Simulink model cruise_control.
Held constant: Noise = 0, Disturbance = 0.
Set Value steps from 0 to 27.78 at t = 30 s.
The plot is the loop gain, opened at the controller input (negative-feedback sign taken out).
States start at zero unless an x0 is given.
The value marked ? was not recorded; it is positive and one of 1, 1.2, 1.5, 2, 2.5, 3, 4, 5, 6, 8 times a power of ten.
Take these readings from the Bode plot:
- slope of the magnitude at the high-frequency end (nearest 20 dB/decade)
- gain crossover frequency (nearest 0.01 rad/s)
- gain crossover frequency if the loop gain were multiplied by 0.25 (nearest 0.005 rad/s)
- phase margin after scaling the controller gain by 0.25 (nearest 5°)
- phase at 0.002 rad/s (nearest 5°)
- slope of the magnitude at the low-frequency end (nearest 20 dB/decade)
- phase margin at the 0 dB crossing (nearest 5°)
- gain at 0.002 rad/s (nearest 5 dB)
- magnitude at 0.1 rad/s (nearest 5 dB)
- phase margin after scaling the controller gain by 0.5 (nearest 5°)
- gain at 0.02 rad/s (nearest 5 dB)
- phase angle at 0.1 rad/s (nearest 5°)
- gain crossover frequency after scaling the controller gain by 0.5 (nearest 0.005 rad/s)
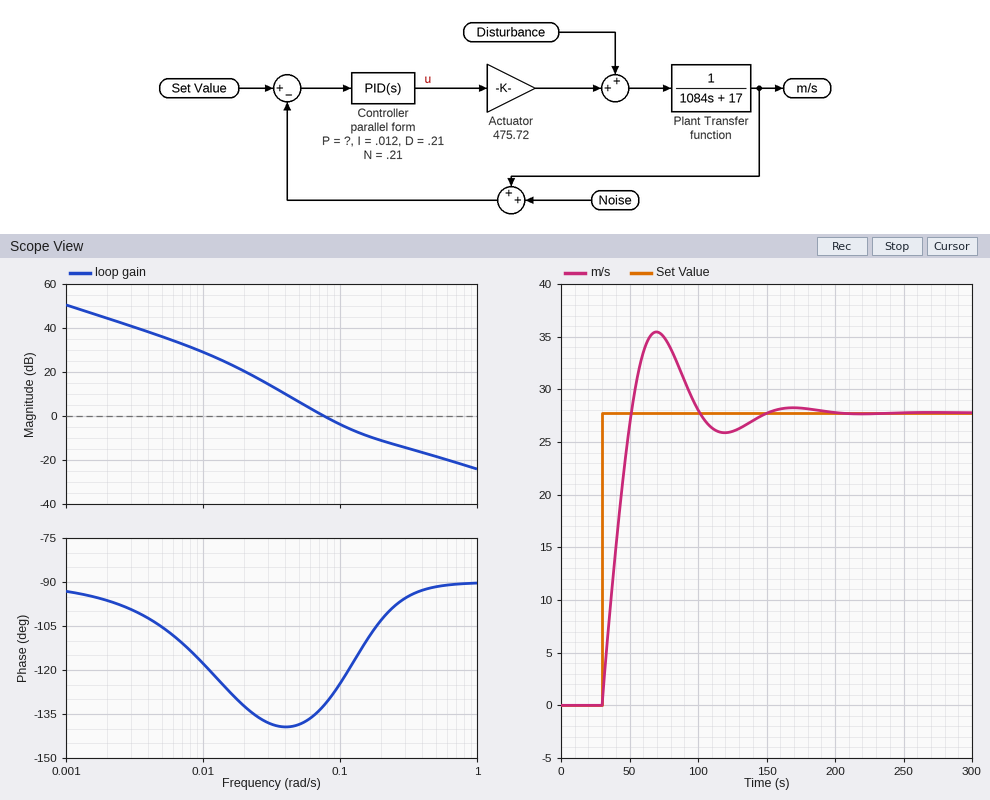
-20 dB/decade
0.08 rad/s
0.035 rad/s
40°
-95°
-20 dB/decade
50°
45 dB
-5 dB
40°
20 dB
-125°
0.050 rad/s
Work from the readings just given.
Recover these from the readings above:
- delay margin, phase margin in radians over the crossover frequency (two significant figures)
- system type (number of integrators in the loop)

11 s
1
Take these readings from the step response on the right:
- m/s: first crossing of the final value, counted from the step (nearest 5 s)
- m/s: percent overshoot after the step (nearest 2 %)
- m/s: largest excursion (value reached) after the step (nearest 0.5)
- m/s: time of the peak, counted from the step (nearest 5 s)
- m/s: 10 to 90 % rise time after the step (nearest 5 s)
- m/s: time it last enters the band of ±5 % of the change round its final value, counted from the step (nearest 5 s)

20 s
28 %
35.5
40 s
15 s
100 s
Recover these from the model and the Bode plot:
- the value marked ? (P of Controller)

0.1
